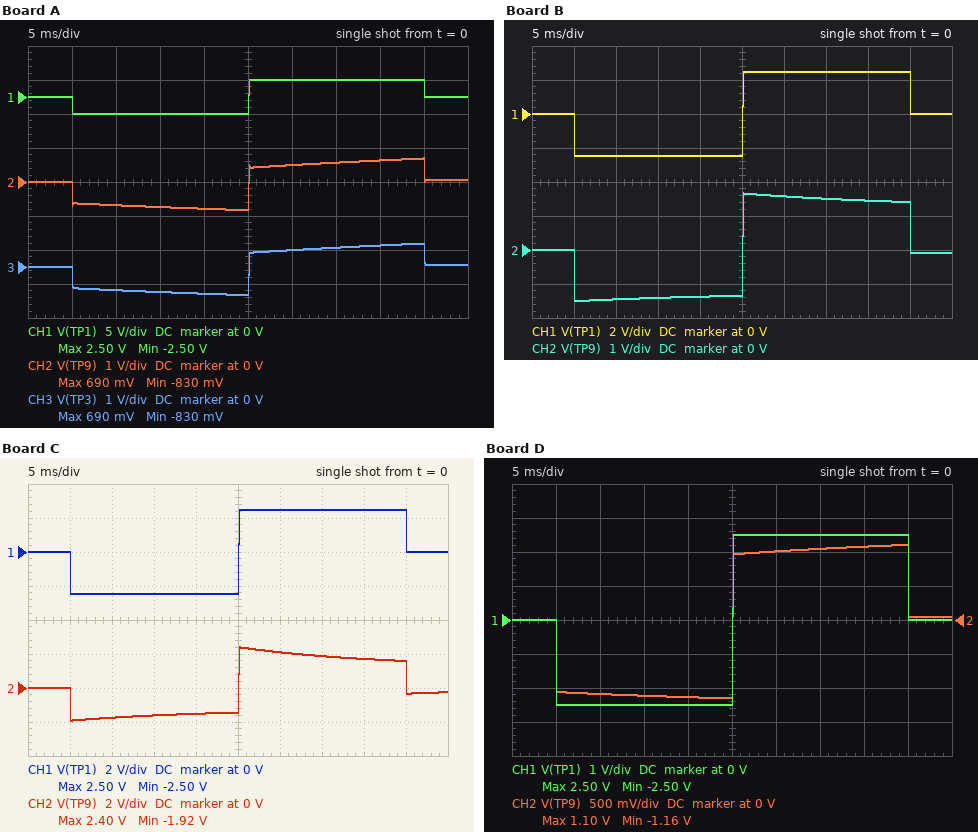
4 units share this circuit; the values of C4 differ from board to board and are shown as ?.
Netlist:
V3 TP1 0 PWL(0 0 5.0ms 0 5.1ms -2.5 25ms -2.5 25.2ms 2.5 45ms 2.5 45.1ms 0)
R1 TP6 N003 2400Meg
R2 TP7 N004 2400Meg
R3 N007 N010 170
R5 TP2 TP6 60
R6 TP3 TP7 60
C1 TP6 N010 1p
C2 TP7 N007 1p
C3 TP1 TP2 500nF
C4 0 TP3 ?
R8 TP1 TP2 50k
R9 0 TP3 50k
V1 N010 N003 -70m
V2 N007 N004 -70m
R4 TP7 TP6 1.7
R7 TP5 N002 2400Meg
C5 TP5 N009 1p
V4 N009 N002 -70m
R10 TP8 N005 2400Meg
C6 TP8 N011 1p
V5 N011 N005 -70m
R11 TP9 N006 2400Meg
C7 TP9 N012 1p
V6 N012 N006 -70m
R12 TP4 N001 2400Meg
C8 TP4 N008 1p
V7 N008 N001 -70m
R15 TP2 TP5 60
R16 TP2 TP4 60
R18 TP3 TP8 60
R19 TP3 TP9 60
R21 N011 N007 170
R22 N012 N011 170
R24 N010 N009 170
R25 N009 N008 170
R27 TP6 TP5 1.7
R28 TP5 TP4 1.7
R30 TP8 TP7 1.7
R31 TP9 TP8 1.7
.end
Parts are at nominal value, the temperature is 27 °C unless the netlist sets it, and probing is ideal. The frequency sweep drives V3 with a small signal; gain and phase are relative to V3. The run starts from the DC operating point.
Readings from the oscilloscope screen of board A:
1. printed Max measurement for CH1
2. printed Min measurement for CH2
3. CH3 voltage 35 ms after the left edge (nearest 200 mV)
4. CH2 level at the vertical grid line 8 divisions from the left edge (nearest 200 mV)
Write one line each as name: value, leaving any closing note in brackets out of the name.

printed Max measurement for CH1: 2.50 V
printed Min measurement for CH2: -830 mV
CH3 voltage 35 ms after the left edge: 600 mV
CH2 level at the vertical grid line 8 divisions from the left edge: 600 mV
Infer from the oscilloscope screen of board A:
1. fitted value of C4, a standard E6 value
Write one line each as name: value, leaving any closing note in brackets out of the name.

fitted value of C4, a standard E6 value: 1.5 µF
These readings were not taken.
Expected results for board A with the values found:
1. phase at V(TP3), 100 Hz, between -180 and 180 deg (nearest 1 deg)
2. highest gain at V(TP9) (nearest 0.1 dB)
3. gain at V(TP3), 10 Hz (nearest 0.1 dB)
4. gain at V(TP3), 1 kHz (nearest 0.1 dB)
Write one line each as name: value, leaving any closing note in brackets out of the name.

phase at V(TP3), 100 Hz, between -180 and 180 deg: -2 deg
highest gain at V(TP9): -6.0 dB
gain at V(TP3), 10 Hz: -11.0 dB
gain at V(TP3), 1 kHz: -12.1 dB
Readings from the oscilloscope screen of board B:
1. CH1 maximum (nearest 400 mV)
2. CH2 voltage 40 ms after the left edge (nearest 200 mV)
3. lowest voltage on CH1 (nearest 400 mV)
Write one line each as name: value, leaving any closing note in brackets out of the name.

CH1 maximum: 2.4 V
CH2 voltage 40 ms after the left edge: 1.4 V
lowest voltage on CH1: -2.4 V
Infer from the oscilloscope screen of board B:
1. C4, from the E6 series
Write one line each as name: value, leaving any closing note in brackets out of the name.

C4, from the E6 series: 330 nF
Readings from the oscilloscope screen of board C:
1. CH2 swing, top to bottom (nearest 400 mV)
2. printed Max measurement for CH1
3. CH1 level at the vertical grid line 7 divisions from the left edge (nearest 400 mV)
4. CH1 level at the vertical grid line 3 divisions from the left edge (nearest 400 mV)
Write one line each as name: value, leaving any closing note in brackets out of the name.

CH2 swing, top to bottom: 4.4 V
printed Max measurement for CH1: 2.50 V
CH1 level at the vertical grid line 7 divisions from the left edge: 2.4 V
CH1 level at the vertical grid line 3 divisions from the left edge: -2.4 V
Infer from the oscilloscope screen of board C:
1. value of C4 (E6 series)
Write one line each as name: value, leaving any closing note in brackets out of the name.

value of C4: 150 nF
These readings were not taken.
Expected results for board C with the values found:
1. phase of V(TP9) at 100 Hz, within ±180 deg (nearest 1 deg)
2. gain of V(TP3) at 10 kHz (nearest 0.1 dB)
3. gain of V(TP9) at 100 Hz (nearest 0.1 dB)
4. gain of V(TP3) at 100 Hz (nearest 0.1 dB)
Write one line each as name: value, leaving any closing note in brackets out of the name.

phase of V(TP9) at 100 Hz, within ±180 deg: 2 deg
gain of V(TP3) at 10 kHz: -2.7 dB
gain of V(TP9) at 100 Hz: -2.3 dB
gain of V(TP3) at 100 Hz: -2.3 dB
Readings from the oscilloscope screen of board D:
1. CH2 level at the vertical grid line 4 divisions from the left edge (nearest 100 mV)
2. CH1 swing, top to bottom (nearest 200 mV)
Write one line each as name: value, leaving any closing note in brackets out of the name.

CH2 level at the vertical grid line 4 divisions from the left edge: -1.1 V
CH1 swing, top to bottom: 5.0 V
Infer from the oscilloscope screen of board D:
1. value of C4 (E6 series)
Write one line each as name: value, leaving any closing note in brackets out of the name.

value of C4: 680 nF
